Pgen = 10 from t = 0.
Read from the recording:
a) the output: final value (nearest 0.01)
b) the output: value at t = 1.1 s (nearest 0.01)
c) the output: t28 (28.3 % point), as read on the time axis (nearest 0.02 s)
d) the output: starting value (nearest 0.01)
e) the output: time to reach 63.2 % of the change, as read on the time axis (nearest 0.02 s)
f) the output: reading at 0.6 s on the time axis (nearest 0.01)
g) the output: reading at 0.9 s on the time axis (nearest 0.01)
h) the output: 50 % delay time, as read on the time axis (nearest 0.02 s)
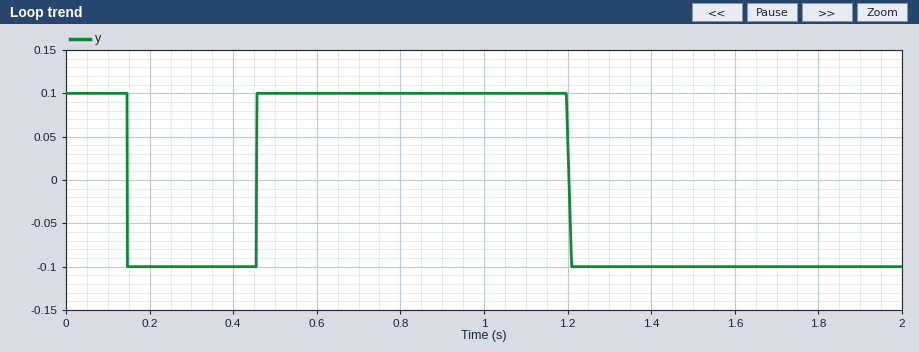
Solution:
-0.10
0.10
0.14 s
0.10
0.14 s
0.10
0.10
0.14 s
